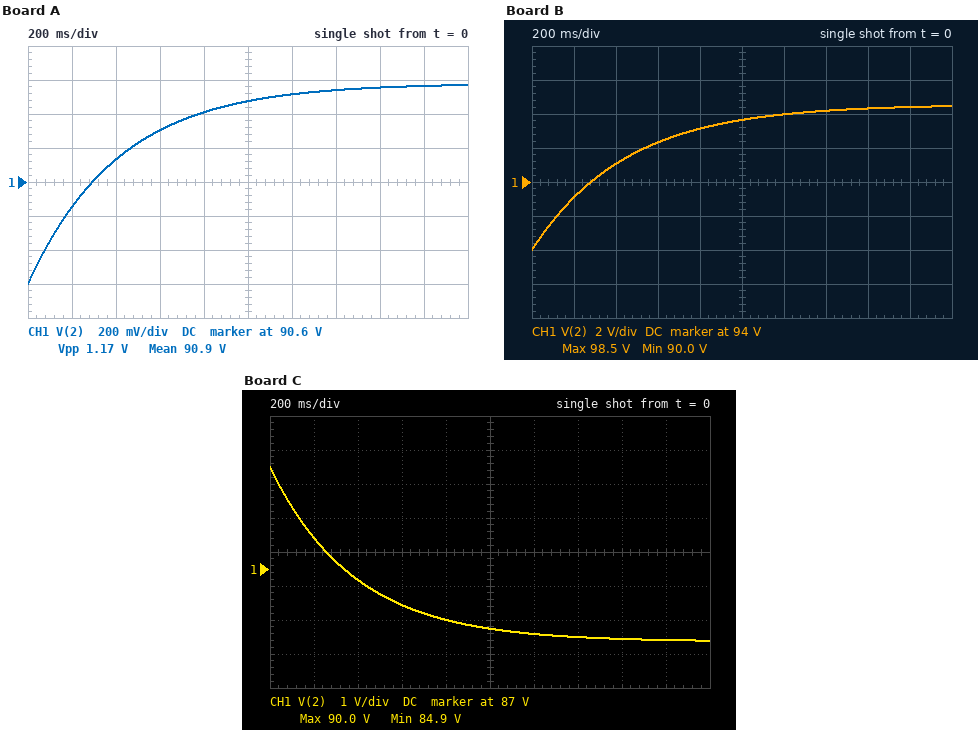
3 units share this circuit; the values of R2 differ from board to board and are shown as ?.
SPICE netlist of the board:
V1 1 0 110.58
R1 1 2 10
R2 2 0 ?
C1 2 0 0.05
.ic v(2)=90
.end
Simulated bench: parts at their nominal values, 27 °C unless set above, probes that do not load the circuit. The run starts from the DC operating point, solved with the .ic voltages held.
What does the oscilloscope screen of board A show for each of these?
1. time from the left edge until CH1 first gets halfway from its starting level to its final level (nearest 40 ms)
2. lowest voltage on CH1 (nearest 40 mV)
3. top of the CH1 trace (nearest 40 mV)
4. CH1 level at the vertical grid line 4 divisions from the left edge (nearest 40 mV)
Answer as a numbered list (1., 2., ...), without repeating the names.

1. 280 ms
2. 90.00 V
3. 91.16 V
4. 91.00 V
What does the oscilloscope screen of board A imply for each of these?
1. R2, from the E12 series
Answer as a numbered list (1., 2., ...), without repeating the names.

1. 47 Ω
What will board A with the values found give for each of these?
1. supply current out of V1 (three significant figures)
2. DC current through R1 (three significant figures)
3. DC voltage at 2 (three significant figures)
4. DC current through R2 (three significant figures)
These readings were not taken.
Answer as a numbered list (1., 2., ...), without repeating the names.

1. 1.94 A
2. 1.94 A
3. 91.2 V
4. 1.94 A
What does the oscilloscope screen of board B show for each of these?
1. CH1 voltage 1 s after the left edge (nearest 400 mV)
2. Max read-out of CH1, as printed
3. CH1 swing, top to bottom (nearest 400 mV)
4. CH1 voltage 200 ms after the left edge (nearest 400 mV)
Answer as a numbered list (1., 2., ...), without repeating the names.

1. 97.6 V
2. 98.5 V
3. 8.4 V
4. 93.2 V
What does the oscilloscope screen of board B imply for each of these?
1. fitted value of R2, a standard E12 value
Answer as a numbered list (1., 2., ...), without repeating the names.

1. 82 Ω
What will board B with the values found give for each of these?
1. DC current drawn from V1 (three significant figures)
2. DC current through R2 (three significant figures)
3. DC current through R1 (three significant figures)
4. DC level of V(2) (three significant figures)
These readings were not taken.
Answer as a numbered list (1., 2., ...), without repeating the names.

1. 1.20 A
2. 1.20 A
3. 1.20 A
4. 98.6 V
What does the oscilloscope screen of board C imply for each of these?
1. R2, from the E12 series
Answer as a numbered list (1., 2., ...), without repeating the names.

1. 33 Ω
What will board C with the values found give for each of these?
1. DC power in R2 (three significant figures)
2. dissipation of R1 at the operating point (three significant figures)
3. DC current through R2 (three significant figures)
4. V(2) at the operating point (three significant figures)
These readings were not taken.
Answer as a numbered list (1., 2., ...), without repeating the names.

1. 218 W
2. 66.1 W
3. 2.57 A
4. 84.9 V
